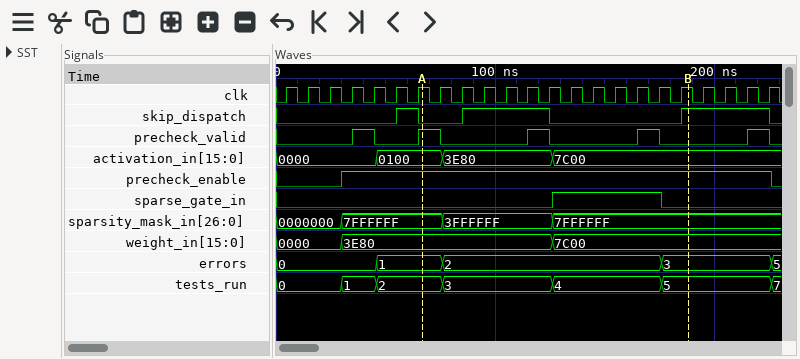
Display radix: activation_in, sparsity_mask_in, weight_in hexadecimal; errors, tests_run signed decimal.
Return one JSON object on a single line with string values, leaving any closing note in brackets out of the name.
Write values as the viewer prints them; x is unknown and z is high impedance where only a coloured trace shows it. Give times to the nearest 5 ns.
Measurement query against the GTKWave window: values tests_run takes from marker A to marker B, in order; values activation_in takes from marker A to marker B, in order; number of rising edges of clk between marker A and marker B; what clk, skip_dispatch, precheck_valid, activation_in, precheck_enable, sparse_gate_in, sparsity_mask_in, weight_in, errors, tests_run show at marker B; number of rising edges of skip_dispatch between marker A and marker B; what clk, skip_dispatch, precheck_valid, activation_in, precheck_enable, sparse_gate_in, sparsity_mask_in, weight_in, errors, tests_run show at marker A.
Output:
{"values tests_run takes from marker A to marker B, in order": "2, 3, 4, 5", "values activation_in takes from marker A to marker B, in order": "0100, 3E80, 7C00", "number of rising edges of clk between marker A and marker B": "12", "what clk, skip_dispatch, precheck_valid, activation_in, precheck_enable, sparse_gate_in, sparsity_mask_in, weight_in, errors, tests_run show at marker B": "clk=1, skip_dispatch=1, precheck_valid=0, activation_in=7C00, precheck_enable=1, sparse_gate_in=0, sparsity_mask_in=7FFFFFF, weight_in=7C00, errors=3, tests_run=5", "number of rising edges of skip_dispatch between marker A and marker B": "2", "what clk, skip_dispatch, precheck_valid, activation_in, precheck_enable, sparse_gate_in, sparsity_mask_in, weight_in, errors, tests_run show at marker A": "clk=1, skip_dispatch=0, precheck_valid=1, activation_in=0100, precheck_enable=1, sparse_gate_in=0, sparsity_mask_in=7FFFFFF, weight_in=3E80, errors=1, tests_run=2"}
